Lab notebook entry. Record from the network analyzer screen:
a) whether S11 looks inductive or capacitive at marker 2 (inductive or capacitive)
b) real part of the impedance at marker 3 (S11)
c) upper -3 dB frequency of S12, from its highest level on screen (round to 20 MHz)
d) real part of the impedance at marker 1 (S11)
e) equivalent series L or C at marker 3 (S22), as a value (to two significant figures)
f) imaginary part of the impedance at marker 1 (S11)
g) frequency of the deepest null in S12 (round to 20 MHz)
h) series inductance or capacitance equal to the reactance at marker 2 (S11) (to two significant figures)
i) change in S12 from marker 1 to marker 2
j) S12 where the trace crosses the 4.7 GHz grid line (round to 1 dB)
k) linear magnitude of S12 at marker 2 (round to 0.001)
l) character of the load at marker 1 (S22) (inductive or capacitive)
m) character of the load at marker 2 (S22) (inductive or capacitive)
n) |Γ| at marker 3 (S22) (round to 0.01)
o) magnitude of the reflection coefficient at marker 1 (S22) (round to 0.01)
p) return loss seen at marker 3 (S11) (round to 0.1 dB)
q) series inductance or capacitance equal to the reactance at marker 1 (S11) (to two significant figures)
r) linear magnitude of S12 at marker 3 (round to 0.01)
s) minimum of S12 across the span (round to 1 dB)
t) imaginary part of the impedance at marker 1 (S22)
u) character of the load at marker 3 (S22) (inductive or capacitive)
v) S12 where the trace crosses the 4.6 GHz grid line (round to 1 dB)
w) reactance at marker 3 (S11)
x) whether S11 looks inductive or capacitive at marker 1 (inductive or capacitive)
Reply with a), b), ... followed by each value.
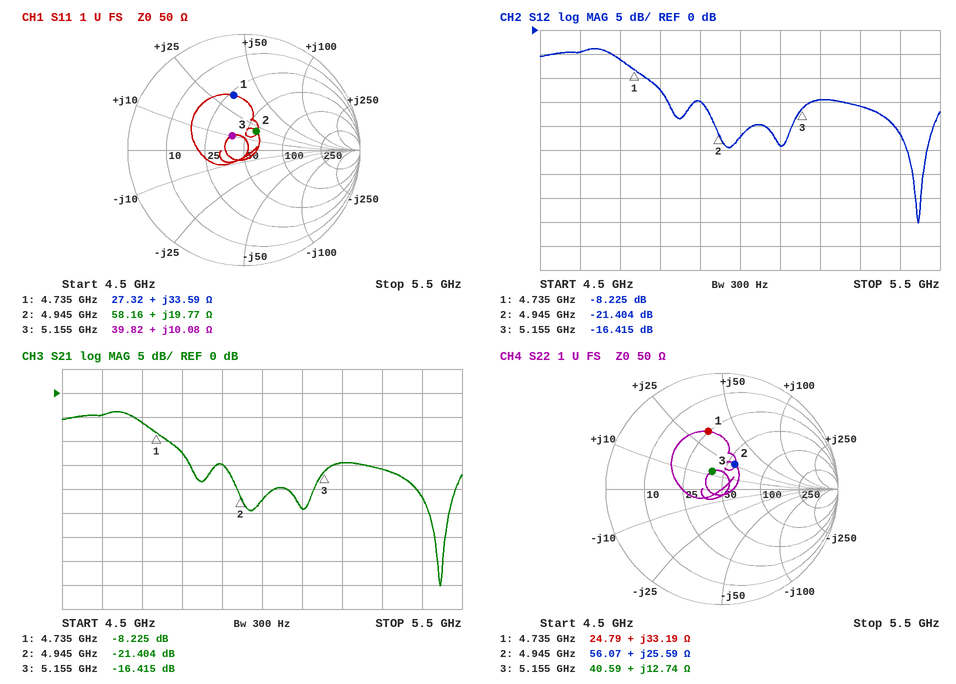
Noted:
a) inductive
b) 39.82 Ω
c) 4.72 GHz
d) 27.32 Ω
e) 390 pH
f) +33.59 Ω
g) 5.44 GHz
h) 640 pH
i) -13.179 dB
j) -6 dB
k) 0.085
l) inductive
m) inductive
n) 0.17
o) 0.51
p) 16.0 dB
q) 1.1 nH
r) 0.15
s) -40 dB
t) +33.19 Ω
u) inductive
v) -5 dB
w) +10.08 Ω
x) inductive
